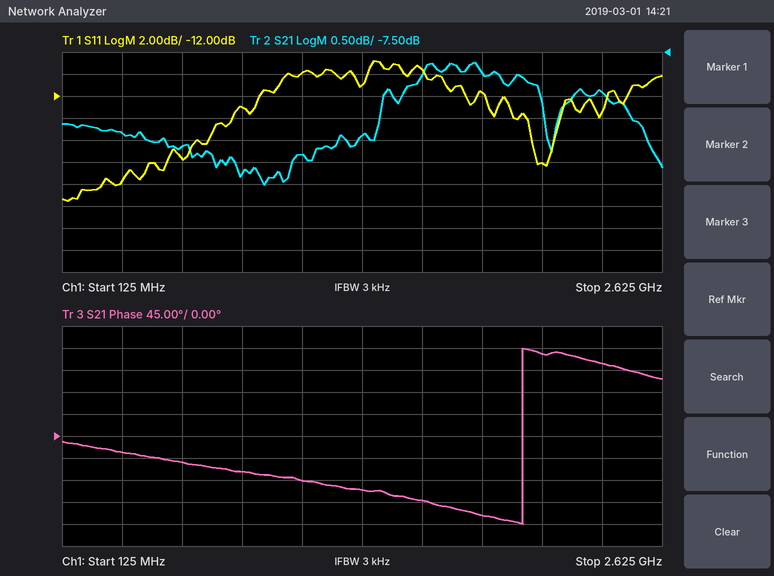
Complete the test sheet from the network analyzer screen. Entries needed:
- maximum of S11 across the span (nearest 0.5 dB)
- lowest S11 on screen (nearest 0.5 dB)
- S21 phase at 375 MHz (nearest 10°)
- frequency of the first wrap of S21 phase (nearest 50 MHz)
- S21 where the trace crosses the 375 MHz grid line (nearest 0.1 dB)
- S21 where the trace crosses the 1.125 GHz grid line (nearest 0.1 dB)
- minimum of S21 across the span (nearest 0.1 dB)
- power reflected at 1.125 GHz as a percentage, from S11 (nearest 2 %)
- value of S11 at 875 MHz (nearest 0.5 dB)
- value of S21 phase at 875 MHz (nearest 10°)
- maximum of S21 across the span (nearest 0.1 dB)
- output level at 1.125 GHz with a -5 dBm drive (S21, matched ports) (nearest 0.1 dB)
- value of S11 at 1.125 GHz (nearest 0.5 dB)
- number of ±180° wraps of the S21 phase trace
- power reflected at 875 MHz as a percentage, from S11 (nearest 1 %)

-9.0 dB
-21.5 dB
-30°
2.05 GHz
-9.3 dB
-9.8 dB
-10.5 dB
10 %
-13.0 dB
-70°
-7.7 dB
-14.8 dBm
-10.0 dB
1
5 %
